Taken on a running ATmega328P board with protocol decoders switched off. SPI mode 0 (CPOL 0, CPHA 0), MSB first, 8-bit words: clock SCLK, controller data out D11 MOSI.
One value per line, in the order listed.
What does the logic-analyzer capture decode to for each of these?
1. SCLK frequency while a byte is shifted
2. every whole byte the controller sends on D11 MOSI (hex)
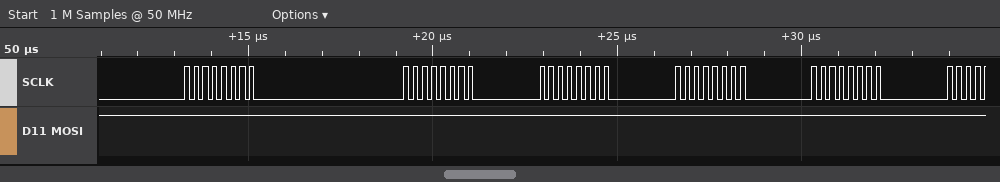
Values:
4 MHz
FF FF FF FF FF
